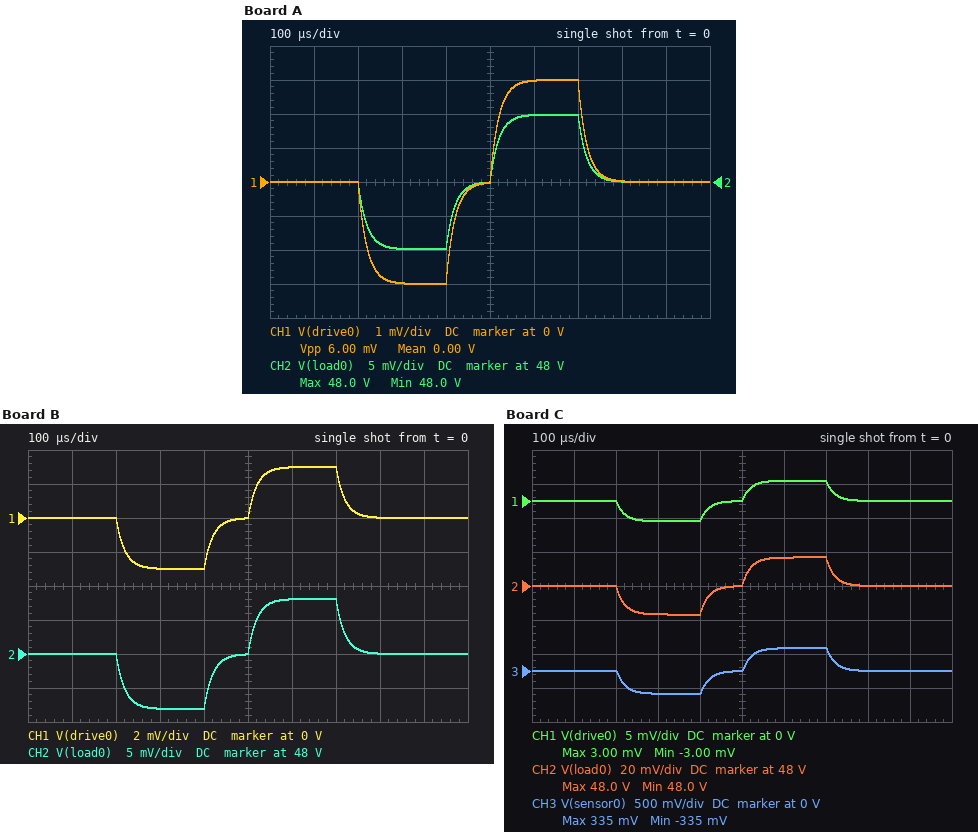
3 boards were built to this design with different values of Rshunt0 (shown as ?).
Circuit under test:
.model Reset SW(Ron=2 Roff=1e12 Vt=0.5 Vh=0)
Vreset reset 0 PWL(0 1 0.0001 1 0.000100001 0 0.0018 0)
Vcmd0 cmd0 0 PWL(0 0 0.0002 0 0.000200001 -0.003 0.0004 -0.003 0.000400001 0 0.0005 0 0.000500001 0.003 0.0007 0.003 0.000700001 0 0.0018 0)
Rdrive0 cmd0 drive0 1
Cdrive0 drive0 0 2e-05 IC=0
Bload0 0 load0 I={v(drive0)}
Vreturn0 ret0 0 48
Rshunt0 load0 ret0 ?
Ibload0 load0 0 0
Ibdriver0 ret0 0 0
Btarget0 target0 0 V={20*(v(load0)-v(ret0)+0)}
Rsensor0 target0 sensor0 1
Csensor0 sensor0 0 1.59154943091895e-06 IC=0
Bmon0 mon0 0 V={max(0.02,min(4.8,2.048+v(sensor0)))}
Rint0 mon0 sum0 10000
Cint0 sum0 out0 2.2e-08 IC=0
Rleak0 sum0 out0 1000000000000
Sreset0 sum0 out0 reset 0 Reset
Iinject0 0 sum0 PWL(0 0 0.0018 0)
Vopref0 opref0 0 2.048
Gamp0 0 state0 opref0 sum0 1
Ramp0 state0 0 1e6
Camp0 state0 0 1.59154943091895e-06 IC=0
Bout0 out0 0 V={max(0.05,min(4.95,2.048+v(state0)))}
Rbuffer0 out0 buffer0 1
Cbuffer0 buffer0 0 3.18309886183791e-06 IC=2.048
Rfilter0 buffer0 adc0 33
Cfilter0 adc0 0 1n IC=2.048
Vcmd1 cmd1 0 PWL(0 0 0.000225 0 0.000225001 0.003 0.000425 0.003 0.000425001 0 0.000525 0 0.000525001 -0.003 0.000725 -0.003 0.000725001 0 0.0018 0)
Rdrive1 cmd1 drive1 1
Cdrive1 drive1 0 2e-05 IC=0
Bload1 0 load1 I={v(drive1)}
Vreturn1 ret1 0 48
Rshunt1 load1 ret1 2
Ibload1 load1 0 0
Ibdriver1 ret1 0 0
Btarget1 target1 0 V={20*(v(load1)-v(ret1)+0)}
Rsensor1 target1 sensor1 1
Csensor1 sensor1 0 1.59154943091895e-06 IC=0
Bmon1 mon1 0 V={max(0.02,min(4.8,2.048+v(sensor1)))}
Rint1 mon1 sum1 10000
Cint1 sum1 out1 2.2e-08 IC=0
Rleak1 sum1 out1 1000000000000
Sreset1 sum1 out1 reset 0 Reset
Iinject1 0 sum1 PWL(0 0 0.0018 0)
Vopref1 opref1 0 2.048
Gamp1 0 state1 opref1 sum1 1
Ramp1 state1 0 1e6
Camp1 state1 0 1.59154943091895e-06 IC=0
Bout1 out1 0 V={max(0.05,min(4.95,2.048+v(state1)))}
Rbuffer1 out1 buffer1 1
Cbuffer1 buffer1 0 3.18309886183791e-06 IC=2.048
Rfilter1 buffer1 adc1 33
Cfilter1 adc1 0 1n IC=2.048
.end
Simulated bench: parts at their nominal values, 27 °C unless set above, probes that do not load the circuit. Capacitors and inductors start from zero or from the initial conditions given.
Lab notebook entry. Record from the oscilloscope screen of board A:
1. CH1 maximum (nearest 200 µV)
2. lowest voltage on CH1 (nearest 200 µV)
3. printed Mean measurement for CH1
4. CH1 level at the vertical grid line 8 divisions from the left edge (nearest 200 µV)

3.0 mV
-3.0 mV
0.00 V
0 V
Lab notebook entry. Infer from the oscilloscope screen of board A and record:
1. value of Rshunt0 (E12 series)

3.3 Ω
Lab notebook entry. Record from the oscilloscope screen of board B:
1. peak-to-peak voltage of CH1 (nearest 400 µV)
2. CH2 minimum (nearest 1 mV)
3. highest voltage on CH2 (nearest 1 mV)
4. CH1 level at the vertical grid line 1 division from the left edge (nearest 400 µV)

6.0 mV
47.992 V
48.008 V
0 V
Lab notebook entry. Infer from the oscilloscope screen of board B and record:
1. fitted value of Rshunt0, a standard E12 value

2.7 Ω
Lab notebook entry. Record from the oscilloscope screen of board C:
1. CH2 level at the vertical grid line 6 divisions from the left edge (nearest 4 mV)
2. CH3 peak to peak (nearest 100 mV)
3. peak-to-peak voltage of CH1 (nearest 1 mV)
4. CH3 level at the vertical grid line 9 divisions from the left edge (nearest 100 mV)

48.016 V
700 mV
6 mV
0 V
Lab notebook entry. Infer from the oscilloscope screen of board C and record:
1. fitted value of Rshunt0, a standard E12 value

5.6 Ω
